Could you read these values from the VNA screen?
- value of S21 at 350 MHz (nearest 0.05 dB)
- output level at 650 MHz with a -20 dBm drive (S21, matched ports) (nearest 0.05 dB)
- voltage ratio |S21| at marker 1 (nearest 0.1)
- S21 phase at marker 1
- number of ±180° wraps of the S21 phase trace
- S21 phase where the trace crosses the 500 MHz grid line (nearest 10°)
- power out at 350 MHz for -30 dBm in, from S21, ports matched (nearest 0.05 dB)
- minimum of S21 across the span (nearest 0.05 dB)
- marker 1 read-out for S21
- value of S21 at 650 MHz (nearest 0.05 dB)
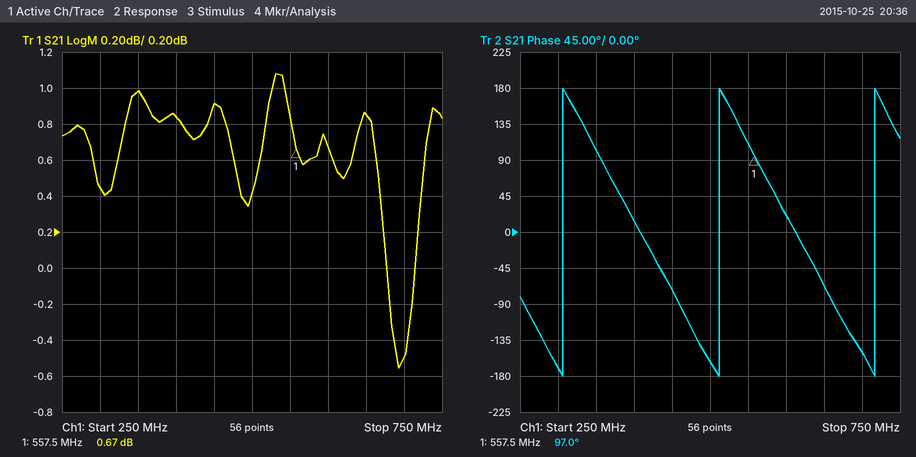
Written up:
1.00 dB
-19.15 dBm
1.1
97.0°
3
-160°
-29.00 dBm
-0.55 dB
0.67 dB
0.85 dB
